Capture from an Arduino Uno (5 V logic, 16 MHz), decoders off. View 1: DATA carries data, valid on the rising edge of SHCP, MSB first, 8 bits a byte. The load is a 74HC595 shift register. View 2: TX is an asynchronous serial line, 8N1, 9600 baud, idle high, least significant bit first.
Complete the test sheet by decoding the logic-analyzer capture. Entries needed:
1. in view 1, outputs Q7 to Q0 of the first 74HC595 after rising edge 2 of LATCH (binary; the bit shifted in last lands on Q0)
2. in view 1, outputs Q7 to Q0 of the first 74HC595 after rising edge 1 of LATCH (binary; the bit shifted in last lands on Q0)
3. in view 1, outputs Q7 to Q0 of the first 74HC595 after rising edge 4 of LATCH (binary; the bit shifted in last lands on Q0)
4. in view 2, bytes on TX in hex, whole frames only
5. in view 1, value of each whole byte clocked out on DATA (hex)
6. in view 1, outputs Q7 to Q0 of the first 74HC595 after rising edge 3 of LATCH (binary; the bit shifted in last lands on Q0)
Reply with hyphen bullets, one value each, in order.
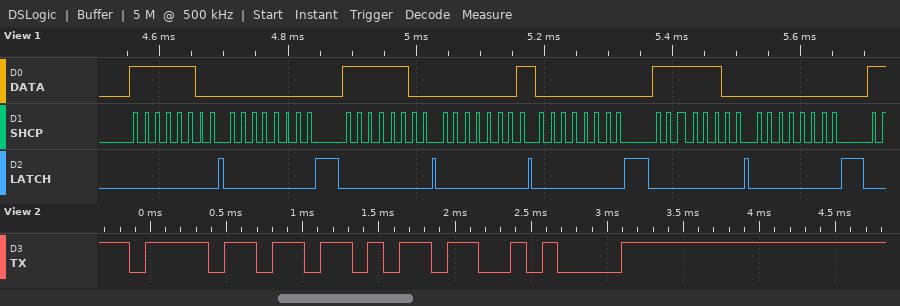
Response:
- 00000000
- 11111100
- 00000001
- 6F 6B 0A
- 0xFC 0x00 0xFC 0x01 0x00 0xFC 0x00
- 11111100
